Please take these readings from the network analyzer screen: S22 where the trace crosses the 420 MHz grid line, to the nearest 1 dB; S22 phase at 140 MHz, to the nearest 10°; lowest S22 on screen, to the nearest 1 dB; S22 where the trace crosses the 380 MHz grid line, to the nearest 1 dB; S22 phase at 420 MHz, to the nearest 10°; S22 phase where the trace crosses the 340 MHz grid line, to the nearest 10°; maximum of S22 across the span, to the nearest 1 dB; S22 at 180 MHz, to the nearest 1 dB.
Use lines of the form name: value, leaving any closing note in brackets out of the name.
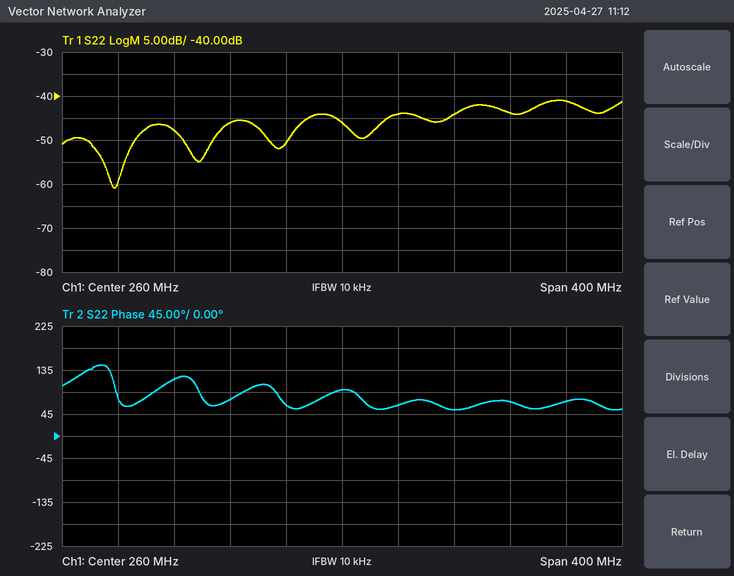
S22 where the trace crosses the 420 MHz grid line, to the nearest 1 dB: -41 dB
S22 phase at 140 MHz, to the nearest 10°: 120°
lowest S22 on screen, to the nearest 1 dB: -61 dB
S22 where the trace crosses the 380 MHz grid line, to the nearest 1 dB: -44 dB
S22 phase at 420 MHz, to the nearest 10°: 70°
S22 phase where the trace crosses the 340 MHz grid line, to the nearest 10°: 50°
maximum of S22 across the span, to the nearest 1 dB: -41 dB
S22 at 180 MHz, to the nearest 1 dB: -46 dB
